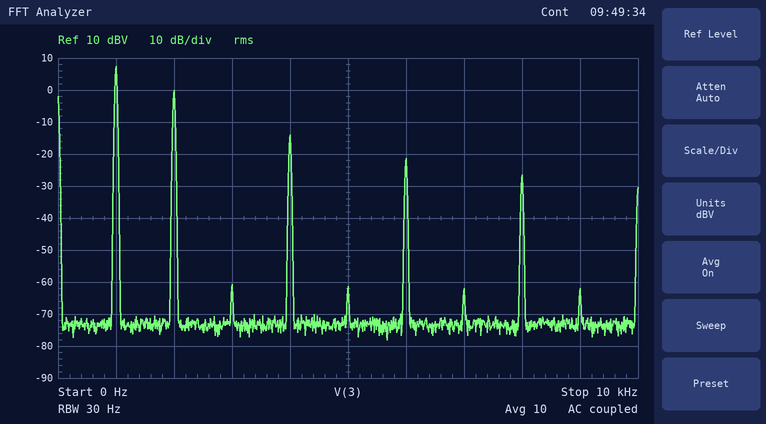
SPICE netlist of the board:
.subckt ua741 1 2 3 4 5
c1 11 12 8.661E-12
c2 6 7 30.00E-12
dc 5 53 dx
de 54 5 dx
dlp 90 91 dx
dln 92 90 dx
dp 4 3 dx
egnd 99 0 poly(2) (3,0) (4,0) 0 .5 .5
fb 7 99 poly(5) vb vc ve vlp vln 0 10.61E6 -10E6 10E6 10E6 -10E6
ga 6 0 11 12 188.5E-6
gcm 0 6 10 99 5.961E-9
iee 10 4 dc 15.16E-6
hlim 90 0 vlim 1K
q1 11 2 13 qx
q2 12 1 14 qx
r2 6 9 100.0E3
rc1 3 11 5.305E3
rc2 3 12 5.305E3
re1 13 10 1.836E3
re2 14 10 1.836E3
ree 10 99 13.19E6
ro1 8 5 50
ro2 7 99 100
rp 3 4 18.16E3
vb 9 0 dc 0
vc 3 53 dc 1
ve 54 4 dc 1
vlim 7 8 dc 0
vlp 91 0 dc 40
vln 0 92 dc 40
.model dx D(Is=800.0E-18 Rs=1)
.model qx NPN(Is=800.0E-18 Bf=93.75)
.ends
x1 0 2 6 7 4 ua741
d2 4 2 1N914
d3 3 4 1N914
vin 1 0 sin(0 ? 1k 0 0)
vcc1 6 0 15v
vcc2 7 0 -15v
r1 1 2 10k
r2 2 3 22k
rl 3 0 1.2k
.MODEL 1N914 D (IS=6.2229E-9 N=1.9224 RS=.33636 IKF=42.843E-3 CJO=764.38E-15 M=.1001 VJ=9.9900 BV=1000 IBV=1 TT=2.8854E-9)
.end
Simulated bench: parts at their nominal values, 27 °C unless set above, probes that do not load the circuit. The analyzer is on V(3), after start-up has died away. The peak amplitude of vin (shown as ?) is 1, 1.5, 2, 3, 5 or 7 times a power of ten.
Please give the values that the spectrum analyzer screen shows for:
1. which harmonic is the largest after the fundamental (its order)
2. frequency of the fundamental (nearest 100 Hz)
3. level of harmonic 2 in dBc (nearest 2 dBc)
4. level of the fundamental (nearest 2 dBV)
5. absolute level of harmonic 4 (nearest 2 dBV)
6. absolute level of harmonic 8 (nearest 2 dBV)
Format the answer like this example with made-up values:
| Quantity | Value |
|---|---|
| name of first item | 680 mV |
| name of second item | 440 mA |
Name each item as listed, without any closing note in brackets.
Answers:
| Quantity | Value |
|---|---|
| which harmonic is the largest after the fundamental | 2 |
| frequency of the fundamental | 1.0 kHz |
| level of harmonic 2 in dBc | -8 dBc |
| level of the fundamental | 8 dBV |
| absolute level of harmonic 4 | -14 dBV |
| absolute level of harmonic 8 | -26 dBV |
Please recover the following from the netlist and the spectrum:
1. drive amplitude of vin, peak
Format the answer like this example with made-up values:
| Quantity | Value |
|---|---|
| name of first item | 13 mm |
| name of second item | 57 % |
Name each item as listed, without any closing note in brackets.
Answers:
| Quantity | Value |
|---|---|
| drive amplitude of vin, peak | 3 V |
